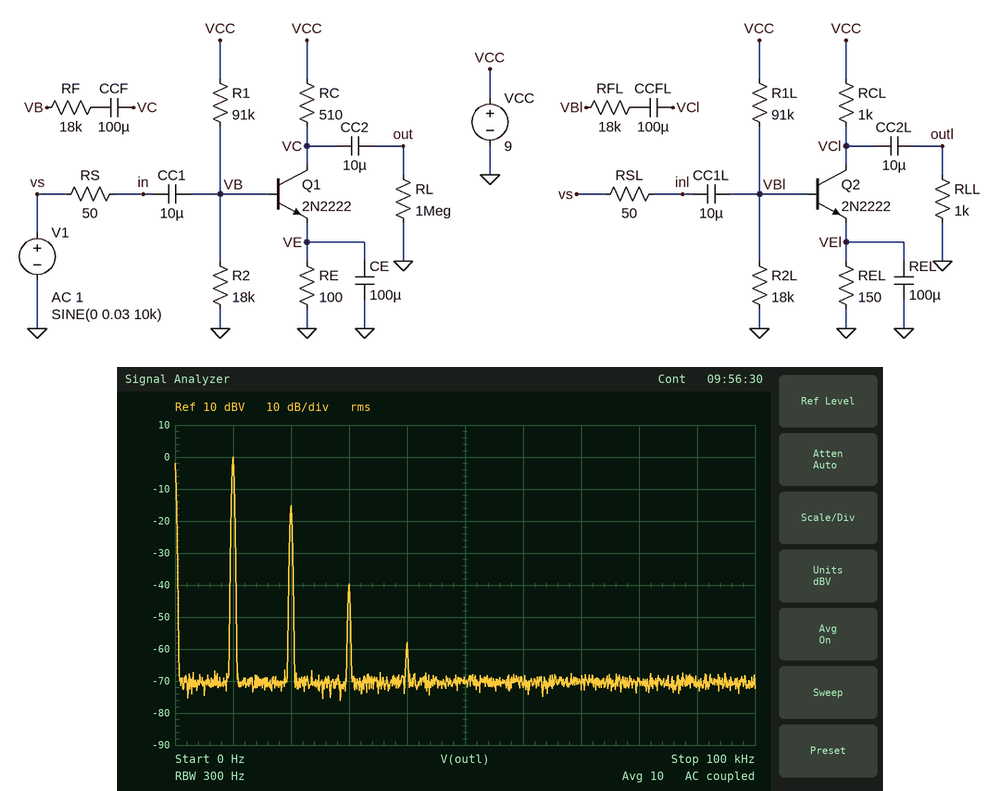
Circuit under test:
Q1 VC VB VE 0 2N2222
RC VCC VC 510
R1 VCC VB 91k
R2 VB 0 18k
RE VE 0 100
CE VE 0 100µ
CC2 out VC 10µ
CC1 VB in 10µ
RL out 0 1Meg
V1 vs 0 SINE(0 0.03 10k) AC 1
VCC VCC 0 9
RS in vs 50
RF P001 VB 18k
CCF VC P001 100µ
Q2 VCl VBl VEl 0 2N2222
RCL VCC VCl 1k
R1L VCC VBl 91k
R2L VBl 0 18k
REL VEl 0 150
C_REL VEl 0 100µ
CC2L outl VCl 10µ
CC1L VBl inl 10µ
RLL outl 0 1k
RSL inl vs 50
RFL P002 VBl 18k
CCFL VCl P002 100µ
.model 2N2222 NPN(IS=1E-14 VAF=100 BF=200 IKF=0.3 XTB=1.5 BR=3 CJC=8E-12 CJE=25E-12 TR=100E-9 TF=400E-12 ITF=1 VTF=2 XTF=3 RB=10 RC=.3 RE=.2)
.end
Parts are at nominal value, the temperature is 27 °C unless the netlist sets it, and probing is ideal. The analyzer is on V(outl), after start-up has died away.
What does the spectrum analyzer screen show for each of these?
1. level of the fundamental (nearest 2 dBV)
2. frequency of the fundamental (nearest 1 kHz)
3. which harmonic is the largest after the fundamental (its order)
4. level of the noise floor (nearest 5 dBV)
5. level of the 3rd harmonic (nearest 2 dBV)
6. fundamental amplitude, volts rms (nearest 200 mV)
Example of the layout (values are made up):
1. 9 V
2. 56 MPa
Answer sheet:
1. 0 dBV
2. 10 kHz
3. 2
4. -70 dBV
5. -40 dBV
6. 1.0 V
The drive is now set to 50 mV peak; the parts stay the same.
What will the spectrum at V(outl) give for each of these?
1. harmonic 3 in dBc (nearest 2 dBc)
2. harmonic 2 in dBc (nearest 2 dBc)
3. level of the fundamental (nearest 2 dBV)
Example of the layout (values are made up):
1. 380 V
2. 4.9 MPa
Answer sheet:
1. -30 dBc
2. -10 dBc
3. 4 dBV
